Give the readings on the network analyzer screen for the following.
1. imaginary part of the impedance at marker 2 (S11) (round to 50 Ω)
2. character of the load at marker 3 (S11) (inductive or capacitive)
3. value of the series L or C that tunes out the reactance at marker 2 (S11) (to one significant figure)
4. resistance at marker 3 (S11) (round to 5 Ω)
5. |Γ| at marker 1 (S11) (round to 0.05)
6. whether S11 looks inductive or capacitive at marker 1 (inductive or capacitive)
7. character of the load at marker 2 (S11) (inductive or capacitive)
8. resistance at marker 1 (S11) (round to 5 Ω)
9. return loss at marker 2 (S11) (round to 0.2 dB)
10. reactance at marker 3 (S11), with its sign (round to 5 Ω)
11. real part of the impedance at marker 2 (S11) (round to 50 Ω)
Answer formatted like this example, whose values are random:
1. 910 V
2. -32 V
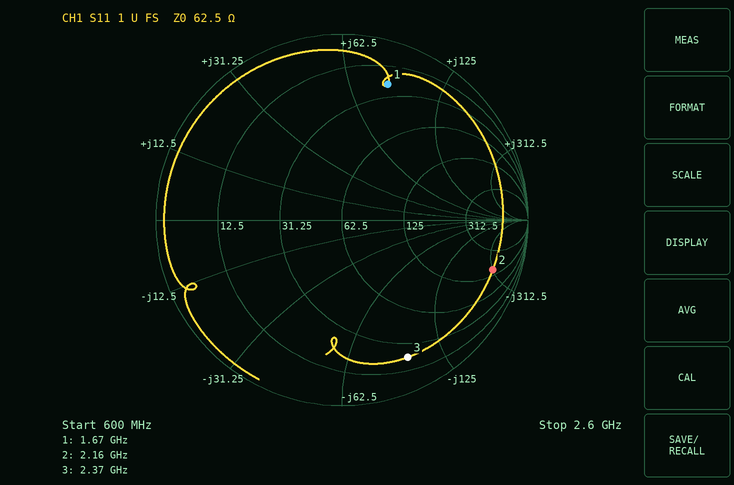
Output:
1. -300 Ω
2. capacitive
3. 20 nH
4. 20 Ω
5. 0.75
6. inductive
7. capacitive
8. 25 Ω
9. 1.4 dB
10. -95 Ω
11. 150 Ω
